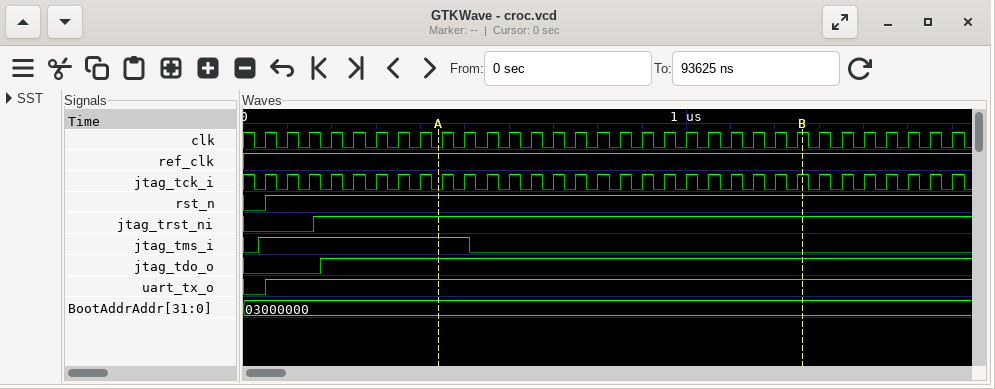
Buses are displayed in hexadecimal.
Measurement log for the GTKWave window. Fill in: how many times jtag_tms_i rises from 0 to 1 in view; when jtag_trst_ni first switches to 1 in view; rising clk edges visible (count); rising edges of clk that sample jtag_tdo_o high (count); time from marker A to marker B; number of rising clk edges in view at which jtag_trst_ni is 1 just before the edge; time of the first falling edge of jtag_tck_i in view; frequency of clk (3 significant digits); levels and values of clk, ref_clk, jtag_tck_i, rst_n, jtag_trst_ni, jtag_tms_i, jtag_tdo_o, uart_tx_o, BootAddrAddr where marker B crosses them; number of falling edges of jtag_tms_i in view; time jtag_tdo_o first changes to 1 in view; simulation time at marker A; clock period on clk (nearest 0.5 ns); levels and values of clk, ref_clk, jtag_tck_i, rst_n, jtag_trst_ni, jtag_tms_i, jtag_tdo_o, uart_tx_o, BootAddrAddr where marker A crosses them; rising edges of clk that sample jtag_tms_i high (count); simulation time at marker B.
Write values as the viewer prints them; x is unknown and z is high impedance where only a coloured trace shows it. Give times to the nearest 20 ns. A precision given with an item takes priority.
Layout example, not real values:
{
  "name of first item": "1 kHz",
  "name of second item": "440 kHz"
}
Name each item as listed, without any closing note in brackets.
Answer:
{
  "how many times jtag_tms_i rises from 0 to 1 in view": "1",
  "when jtag_trst_ni first switches to 1 in view": "160 ns",
  "rising clk edges visible": "32",
  "rising edges of clk that sample jtag_tdo_o high": "29",
  "time from marker A to marker B": "820 ns",
  "number of rising clk edges in view at which jtag_trst_ni is 1 just before the edge": "29",
  "time of the first falling edge of jtag_tck_i in view": "20 ns",
  "frequency of clk": "20.0 MHz",
  "levels and values of clk, ref_clk, jtag_tck_i, rst_n, jtag_trst_ni, jtag_tms_i, jtag_tdo_o, uart_tx_o, BootAddrAddr where marker B crosses them": "clk=1, ref_clk=1, jtag_tck_i=1, rst_n=1, jtag_trst_ni=1, jtag_tms_i=0, jtag_tdo_o=1, uart_tx_o=1, BootAddrAddr=03000000",
  "number of falling edges of jtag_tms_i in view": "1",
  "time jtag_tdo_o first changes to 1 in view": "180 ns",
  "simulation time at marker A": "440 ns",
  "clock period on clk": "50 ns",
  "levels and values of clk, ref_clk, jtag_tck_i, rst_n, jtag_trst_ni, jtag_tms_i, jtag_tdo_o, uart_tx_o, BootAddrAddr where marker A crosses them": "clk=0, ref_clk=1, jtag_tck_i=0, rst_n=1, jtag_trst_ni=1, jtag_tms_i=1, jtag_tdo_o=1, uart_tx_o=1, BootAddrAddr=03000000",
  "rising edges of clk that sample jtag_tms_i high": "10",
  "simulation time at marker B": "1260 ns"
}
